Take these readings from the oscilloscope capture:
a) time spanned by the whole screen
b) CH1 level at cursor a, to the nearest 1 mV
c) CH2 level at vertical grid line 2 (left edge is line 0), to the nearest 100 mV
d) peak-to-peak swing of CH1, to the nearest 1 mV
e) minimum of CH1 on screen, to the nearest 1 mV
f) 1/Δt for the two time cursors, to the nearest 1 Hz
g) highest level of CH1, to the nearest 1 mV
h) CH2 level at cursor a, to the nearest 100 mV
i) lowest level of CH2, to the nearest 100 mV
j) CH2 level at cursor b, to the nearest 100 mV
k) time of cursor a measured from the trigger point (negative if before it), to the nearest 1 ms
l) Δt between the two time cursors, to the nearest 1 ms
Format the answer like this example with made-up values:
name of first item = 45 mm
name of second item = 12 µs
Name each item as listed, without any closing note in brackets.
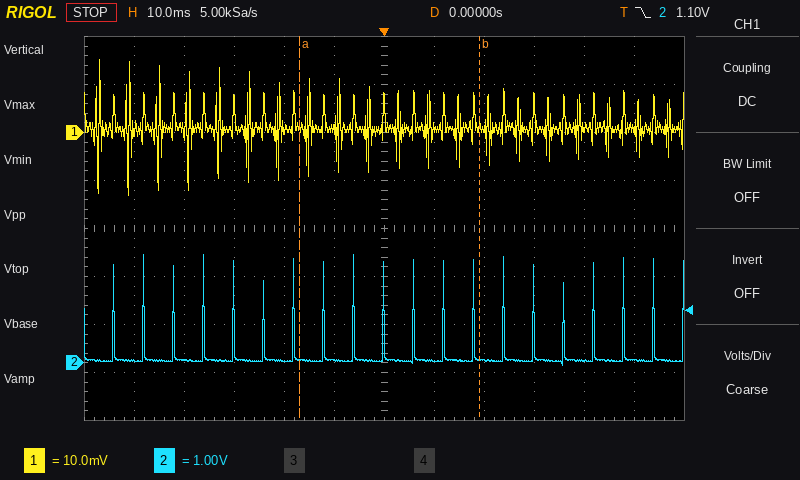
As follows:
time spanned by the whole screen = 120 ms
CH1 level at cursor a, to the nearest 1 mV = 1 mV
CH2 level at vertical grid line 2 (left edge is line 0), to the nearest 100 mV = 100 mV
peak-to-peak swing of CH1, to the nearest 1 mV = 28 mV
minimum of CH1 on screen, to the nearest 1 mV = -13 mV
1/Δt for the two time cursors, to the nearest 1 Hz = 28 Hz
highest level of CH1, to the nearest 1 mV = 15 mV
CH2 level at cursor a, to the nearest 100 mV = 100 mV
lowest level of CH2, to the nearest 100 mV = -100 mV
CH2 level at cursor b, to the nearest 100 mV = 100 mV
time of cursor a measured from the trigger point (negative if before it), to the nearest 1 ms = -17 ms
Δt between the two time cursors, to the nearest 1 ms = 36 ms
